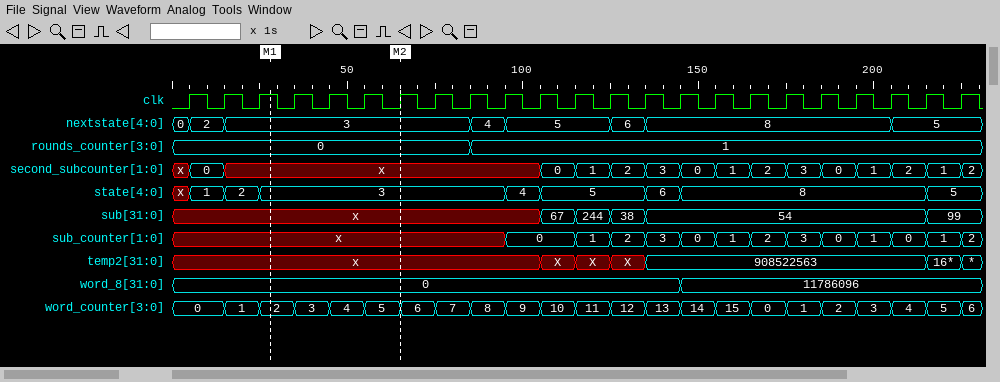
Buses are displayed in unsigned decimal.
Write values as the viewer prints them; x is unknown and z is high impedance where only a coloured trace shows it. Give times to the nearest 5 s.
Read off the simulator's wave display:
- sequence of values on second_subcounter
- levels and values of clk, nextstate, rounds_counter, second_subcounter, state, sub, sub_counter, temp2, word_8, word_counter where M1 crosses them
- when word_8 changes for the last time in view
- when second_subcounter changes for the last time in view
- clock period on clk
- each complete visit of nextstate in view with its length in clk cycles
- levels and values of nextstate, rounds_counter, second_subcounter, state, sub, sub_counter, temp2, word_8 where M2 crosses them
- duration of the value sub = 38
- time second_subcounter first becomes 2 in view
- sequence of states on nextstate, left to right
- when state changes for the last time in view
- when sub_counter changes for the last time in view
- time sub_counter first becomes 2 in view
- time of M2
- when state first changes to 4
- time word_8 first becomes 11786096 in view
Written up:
x, 0, x, 0, 1, 2, 3, 0, 1, 2, 3, 0, 1, 2, 1, 2
clk=1, nextstate=3, rounds_counter=0, second_subcounter=x, state=3, sub=x, sub_counter=x, temp2=x, word_8=0, word_counter=2
145 s
225 s
10 s
2: 1, 3: 7, 4: 1, 5: 3, 6: 1, 8: 7
nextstate=3, rounds_counter=0, second_subcounter=x, state=3, sub=x, sub_counter=x, temp2=x, word_8=0
10 s
125 s
0, 2, 3, 4, 5, 6, 8, 5
215 s
225 s
125 s
65 s
95 s
145 s
